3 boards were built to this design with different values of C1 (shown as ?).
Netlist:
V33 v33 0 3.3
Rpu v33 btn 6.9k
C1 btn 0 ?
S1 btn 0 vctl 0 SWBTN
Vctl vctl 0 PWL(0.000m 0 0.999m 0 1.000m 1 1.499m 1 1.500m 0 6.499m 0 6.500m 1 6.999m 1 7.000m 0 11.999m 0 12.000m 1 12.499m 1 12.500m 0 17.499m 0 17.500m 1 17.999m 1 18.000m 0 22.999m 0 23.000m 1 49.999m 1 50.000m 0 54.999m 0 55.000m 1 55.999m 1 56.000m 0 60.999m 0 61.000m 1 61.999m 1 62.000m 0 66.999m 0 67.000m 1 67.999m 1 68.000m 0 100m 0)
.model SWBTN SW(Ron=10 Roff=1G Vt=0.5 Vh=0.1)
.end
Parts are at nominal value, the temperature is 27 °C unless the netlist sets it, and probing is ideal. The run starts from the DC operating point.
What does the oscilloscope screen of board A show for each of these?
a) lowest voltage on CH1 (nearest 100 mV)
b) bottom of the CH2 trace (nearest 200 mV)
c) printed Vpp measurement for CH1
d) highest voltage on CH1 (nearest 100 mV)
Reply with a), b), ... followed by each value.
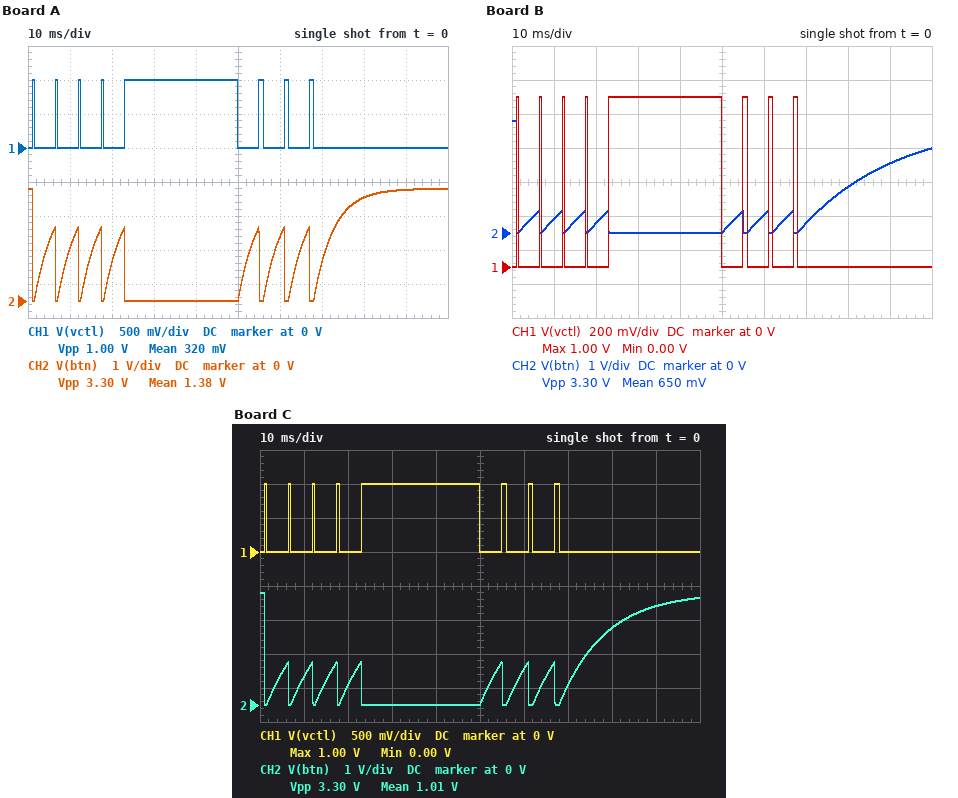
a) 0 V
b) 0 V
c) 1.00 V
d) 1.0 V
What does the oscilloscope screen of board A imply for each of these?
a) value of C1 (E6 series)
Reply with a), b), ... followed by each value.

a) 680 nF
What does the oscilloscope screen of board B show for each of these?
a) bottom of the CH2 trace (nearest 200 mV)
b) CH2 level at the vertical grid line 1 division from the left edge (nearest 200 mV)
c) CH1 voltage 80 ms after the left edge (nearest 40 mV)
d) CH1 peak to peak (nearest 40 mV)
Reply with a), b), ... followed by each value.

a) 0 V
b) 400 mV
c) 0 V
d) 1.00 V
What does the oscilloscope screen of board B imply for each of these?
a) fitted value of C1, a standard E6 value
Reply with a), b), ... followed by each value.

a) 3.3 µF
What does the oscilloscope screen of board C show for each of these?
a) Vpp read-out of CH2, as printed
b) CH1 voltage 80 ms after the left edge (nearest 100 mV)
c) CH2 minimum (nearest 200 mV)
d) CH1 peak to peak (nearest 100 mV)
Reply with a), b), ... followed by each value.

a) 3.30 V
b) 0 V
c) 0 V
d) 1.0 V
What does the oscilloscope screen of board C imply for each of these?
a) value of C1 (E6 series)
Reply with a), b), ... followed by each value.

a) 1.5 µF
